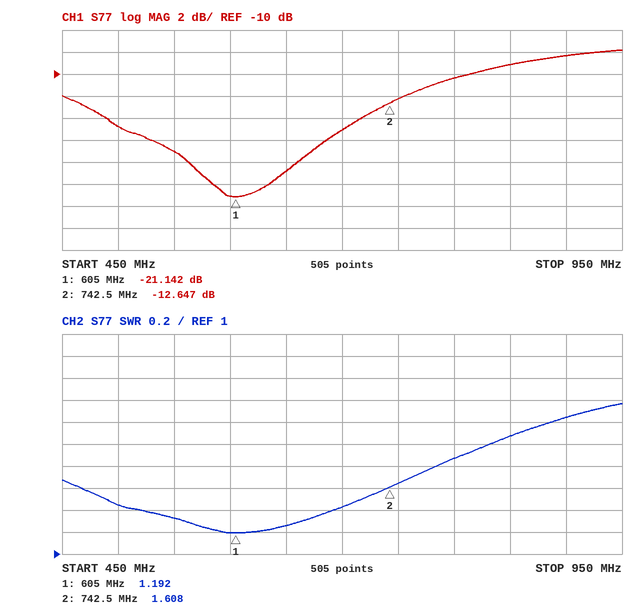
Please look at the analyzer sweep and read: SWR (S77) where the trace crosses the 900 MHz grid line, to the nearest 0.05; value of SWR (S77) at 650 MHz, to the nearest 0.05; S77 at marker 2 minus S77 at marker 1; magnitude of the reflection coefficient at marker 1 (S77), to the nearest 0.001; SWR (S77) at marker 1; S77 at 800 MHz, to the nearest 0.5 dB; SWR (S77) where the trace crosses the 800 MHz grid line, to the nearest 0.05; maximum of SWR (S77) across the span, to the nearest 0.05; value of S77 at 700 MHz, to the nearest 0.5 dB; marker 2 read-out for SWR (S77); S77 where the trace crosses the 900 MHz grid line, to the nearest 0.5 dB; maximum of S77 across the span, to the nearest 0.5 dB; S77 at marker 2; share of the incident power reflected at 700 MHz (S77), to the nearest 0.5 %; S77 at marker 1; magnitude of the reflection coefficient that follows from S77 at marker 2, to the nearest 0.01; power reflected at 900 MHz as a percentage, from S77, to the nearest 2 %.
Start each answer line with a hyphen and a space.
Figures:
- 2.25
- 1.25
- 8.495 dB
- 0.088
- 1.192
- -10.5 dB
- 1.85
- 2.35
- -15.0 dB
- 1.608
- -8.5 dB
- -8.0 dB
- -12.647 dB
- 3.0 %
- -21.142 dB
- 0.23
- 14 %
